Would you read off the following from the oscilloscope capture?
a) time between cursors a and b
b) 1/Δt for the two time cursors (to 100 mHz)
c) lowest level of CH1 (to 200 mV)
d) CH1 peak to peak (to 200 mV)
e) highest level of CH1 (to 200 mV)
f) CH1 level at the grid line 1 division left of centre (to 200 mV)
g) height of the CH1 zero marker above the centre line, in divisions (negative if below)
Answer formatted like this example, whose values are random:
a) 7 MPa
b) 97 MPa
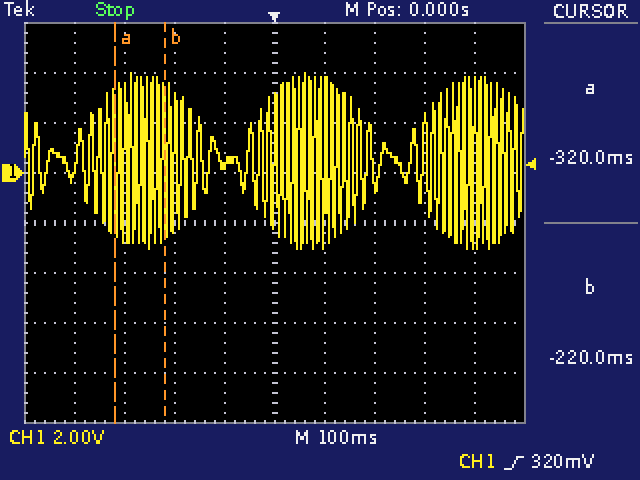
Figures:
a) 100 ms
b) 10.0 Hz
c) -3.0 V
d) 7.0 V
e) 4.0 V
f) 400 mV
g) +1.0 div
